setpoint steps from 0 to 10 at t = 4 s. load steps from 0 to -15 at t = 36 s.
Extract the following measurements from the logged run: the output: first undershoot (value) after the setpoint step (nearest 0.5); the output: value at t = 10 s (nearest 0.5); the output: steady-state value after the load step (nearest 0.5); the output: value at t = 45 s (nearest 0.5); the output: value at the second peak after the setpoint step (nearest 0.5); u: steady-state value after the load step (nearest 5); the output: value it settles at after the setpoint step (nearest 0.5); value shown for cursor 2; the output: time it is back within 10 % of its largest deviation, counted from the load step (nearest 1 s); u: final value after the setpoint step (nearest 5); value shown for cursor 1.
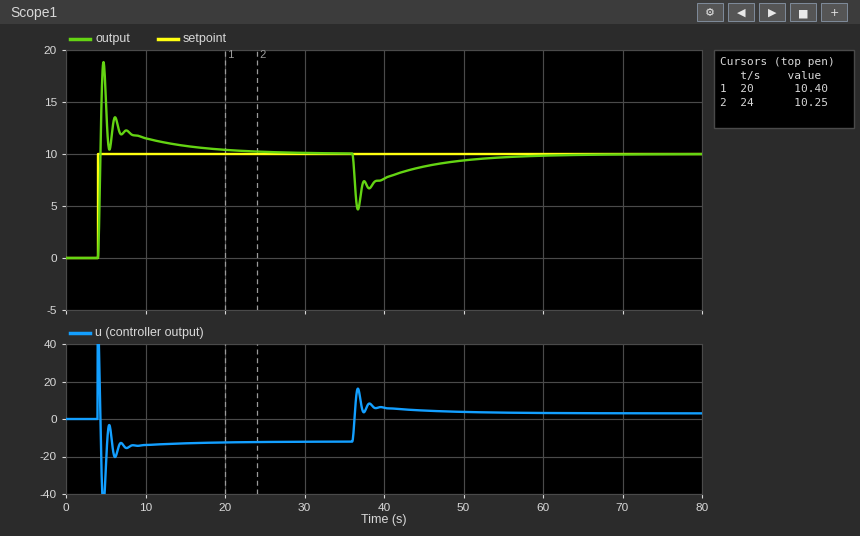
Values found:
10.5
11.5
10.0
9.0
13.5
5
10.0
10.25
15 s
-10
10.40
